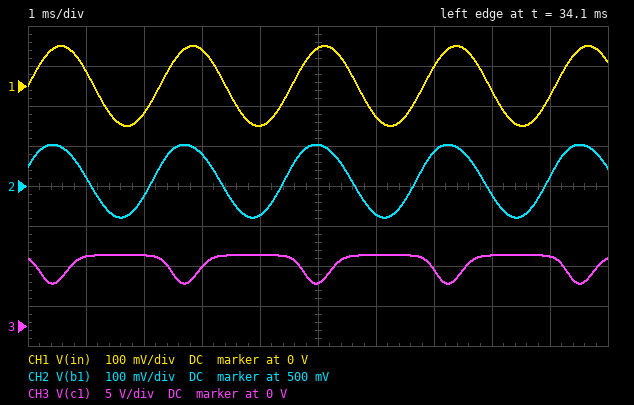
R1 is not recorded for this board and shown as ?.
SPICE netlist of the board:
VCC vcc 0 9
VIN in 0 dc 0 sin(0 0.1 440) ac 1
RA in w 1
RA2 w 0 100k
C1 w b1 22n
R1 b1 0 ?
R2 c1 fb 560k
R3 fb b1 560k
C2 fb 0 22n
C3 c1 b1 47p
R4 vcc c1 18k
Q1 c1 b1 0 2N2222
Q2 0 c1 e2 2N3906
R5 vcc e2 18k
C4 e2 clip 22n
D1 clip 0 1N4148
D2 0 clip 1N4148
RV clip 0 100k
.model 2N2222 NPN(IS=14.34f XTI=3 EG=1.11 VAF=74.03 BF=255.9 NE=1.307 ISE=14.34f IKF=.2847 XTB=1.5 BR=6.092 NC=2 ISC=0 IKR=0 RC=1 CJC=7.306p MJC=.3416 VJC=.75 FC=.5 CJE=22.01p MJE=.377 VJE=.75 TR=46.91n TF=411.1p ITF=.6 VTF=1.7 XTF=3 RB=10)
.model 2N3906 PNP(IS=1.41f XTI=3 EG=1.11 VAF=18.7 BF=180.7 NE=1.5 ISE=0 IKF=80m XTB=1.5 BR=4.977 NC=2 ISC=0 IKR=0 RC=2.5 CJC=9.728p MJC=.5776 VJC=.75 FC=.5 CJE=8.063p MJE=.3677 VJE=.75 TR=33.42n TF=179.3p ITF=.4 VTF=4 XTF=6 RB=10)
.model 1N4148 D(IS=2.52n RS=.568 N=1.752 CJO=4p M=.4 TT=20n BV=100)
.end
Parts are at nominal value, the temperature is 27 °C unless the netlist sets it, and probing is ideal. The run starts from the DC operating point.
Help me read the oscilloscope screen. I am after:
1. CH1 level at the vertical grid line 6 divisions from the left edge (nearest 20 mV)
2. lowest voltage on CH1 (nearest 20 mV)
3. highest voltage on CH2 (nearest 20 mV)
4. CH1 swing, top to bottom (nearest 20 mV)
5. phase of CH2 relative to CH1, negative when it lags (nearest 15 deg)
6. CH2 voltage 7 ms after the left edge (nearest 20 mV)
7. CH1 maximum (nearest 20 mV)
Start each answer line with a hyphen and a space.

- -80 mV
- -100 mV
- 600 mV
- 200 mV
- 15 deg
- 580 mV
- 100 mV
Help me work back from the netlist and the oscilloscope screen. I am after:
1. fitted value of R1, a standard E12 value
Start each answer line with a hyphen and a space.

- 82 kΩ
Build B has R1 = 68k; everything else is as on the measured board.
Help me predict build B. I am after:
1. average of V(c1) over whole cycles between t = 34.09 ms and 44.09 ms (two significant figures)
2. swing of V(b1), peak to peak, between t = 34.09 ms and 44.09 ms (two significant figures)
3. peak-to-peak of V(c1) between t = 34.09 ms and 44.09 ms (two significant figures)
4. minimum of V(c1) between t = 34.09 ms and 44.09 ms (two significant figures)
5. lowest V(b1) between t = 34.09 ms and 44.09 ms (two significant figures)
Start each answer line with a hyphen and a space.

- 8.6 V
- 190 mV
- 1.2 V
- 7.6 V
- 390 mV
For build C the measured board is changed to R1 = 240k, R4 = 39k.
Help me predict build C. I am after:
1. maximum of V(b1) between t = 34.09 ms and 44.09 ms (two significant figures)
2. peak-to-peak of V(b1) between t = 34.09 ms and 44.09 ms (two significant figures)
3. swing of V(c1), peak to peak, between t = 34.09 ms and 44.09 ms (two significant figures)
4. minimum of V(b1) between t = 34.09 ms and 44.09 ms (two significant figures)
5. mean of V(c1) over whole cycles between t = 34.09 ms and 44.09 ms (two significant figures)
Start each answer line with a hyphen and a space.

- 610 mV
- 130 mV
- 8.5 V
- 480 mV
- 5.0 V
